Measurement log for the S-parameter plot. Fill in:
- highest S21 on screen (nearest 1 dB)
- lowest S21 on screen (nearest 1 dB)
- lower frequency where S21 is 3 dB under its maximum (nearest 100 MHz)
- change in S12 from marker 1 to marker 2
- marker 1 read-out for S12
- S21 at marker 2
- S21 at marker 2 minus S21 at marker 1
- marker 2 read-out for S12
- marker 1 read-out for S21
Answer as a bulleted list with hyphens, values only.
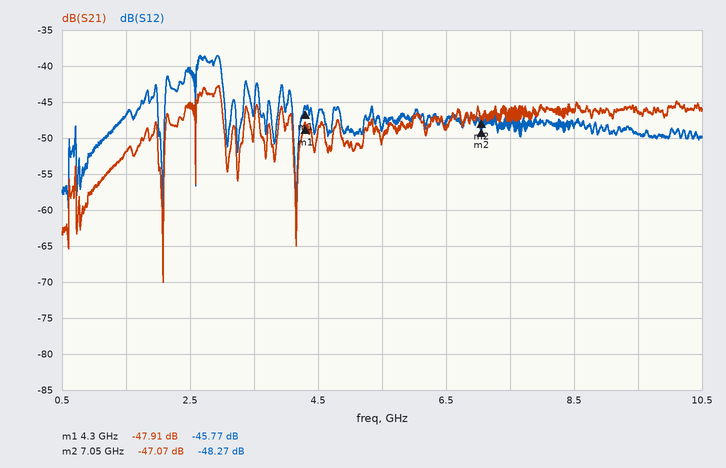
- -43 dB
- -70 dB
- 2.6 GHz
- -2.50 dB
- -45.77 dB
- -47.07 dB
- 0.84 dB
- -48.27 dB
- -47.91 dB
